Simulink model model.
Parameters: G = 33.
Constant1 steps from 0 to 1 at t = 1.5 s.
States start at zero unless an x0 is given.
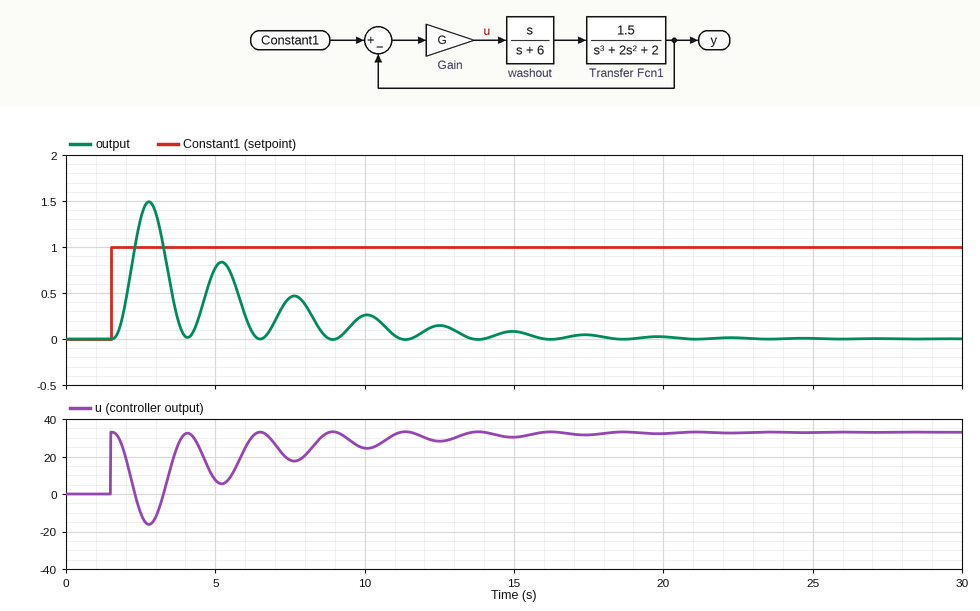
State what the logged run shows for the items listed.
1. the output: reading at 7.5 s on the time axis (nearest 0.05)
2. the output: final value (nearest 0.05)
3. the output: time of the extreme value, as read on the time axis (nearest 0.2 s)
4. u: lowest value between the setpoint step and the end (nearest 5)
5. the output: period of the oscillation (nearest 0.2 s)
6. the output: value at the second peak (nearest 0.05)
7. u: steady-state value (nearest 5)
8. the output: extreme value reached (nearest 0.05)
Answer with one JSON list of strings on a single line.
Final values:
["0.45", "0.00", "2.8 s", "-15", "2.4 s", "0.85", "35", "1.50"]
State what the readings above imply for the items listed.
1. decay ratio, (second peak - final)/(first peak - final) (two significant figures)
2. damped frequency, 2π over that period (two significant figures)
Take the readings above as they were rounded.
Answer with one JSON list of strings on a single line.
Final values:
["0.57", "2.6 rad/s"]
